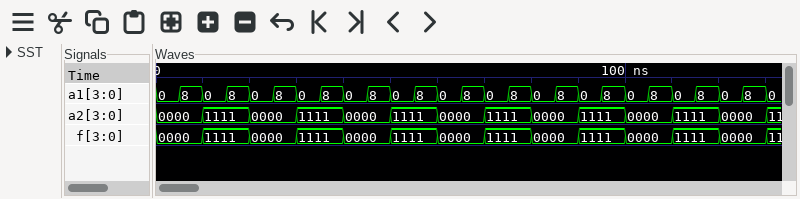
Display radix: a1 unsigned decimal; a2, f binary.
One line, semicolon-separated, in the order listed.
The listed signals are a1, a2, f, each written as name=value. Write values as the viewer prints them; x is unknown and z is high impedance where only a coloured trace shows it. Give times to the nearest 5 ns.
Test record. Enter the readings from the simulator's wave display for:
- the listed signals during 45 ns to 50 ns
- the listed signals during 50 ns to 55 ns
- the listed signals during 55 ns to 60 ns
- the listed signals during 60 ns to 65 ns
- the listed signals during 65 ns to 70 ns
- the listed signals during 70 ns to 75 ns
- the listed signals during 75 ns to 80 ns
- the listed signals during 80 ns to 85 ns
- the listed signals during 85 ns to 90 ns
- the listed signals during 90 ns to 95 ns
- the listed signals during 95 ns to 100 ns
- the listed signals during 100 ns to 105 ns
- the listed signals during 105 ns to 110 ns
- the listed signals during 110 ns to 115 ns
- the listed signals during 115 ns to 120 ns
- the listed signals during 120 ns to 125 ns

a1=8, a2=0000, f=0000; a1=0, a2=1111, f=1111; a1=8, a2=1111, f=1111; a1=0, a2=0000, f=0000; a1=8, a2=0000, f=0000; a1=0, a2=1111, f=1111; a1=8, a2=1111, f=1111; a1=0, a2=0000, f=0000; a1=8, a2=0000, f=0000; a1=0, a2=1111, f=1111; a1=8, a2=1111, f=1111; a1=0, a2=0000, f=0000; a1=8, a2=0000, f=0000; a1=0, a2=1111, f=1111; a1=8, a2=1111, f=1111; a1=0, a2=0000, f=0000
